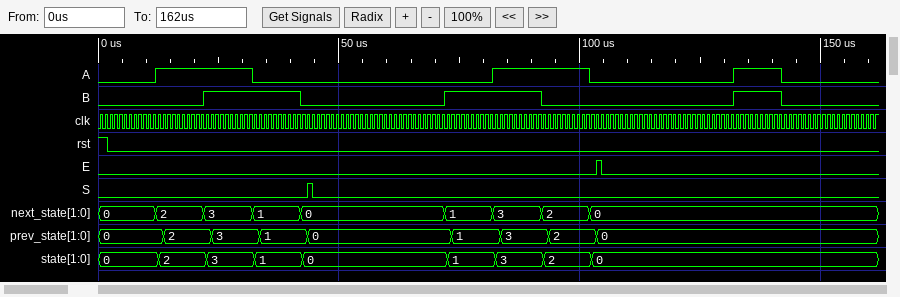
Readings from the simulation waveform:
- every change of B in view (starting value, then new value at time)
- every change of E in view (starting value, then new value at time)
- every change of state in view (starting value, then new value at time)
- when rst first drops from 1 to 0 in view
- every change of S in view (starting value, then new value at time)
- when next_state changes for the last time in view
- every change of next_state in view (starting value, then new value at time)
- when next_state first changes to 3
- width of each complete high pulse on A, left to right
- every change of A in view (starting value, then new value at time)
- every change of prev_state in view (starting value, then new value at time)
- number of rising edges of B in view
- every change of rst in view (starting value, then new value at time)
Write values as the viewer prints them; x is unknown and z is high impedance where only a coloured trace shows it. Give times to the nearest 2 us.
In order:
0, 1 at 22 us, 0 at 42 us, 1 at 72 us, 0 at 92 us, 1 at 132 us, 0 at 142 us
0, 1 at 104 us, 0 at 104 us
0, 2 at 12 us, 3 at 22 us, 1 at 32 us, 0 at 42 us, 1 at 72 us, 3 at 82 us, 2 at 92 us, 0 at 102 us
2 us
0, 1 at 44 us, 0 at 44 us
102 us
0, 2 at 12 us, 3 at 22 us, 1 at 32 us, 0 at 42 us, 1 at 72 us, 3 at 82 us, 2 at 92 us, 0 at 102 us
22 us
20 us, 20 us, 10 us
0, 1 at 12 us, 0 at 32 us, 1 at 82 us, 0 at 102 us, 1 at 132 us, 0 at 142 us
0, 2 at 14 us, 3 at 24 us, 1 at 34 us, 0 at 44 us, 1 at 74 us, 3 at 84 us, 2 at 94 us, 0 at 104 us
3
1, 0 at 2 us
